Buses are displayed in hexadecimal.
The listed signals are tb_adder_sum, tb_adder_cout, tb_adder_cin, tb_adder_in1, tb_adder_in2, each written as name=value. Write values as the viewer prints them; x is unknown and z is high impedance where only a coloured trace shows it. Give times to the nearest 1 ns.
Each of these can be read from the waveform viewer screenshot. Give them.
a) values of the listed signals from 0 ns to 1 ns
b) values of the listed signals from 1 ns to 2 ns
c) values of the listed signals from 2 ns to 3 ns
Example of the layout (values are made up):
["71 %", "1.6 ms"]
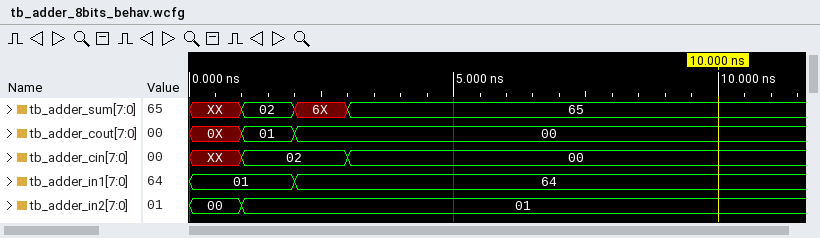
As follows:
["tb_adder_sum=XX, tb_adder_cout=0X, tb_adder_cin=XX, tb_adder_in1=01, tb_adder_in2=00", "tb_adder_sum=02, tb_adder_cout=01, tb_adder_cin=02, tb_adder_in1=01, tb_adder_in2=01", "tb_adder_sum=6X, tb_adder_cout=00, tb_adder_cin=02, tb_adder_in1=64, tb_adder_in2=01"]
